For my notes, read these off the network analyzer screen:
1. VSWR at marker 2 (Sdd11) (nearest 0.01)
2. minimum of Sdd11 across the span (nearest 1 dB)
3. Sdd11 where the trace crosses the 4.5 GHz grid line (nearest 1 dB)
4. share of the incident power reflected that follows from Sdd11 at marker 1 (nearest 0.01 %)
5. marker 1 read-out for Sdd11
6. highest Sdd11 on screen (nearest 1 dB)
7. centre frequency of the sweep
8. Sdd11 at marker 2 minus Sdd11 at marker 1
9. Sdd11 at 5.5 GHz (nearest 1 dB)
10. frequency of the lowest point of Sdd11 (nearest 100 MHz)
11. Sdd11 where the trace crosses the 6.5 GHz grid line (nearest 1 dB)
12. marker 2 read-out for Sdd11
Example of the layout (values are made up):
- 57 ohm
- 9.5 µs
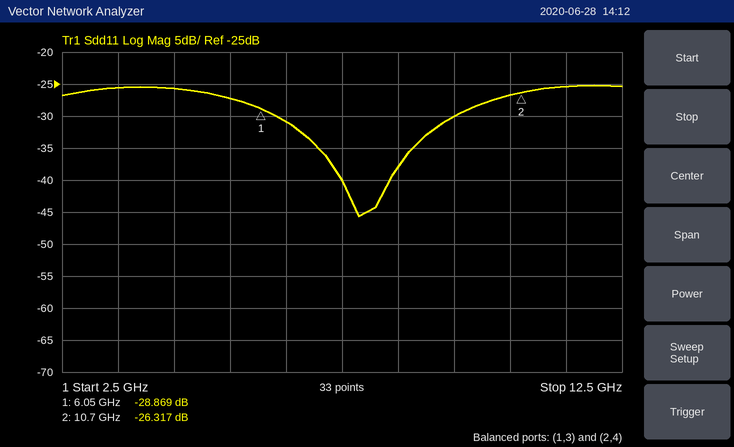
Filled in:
- 1.10
- -46 dB
- -26 dB
- 0.13 %
- -28.869 dB
- -25 dB
- 7.5 GHz
- 2.552 dB
- -27 dB
- 7.8 GHz
- -31 dB
- -26.317 dB
